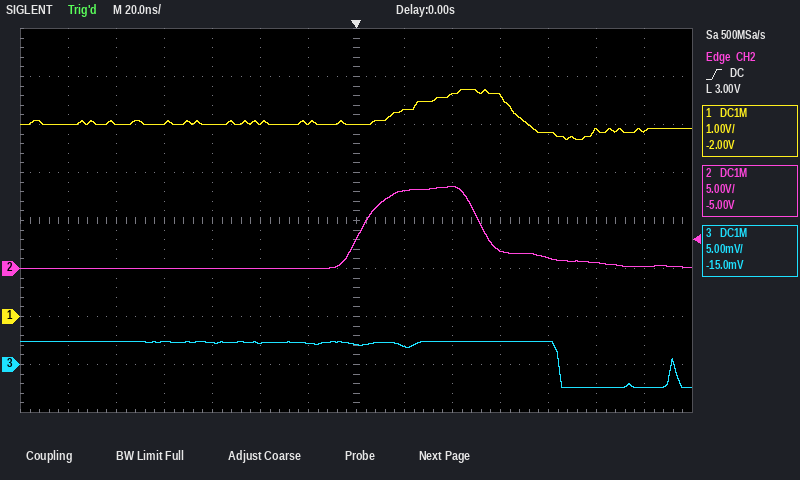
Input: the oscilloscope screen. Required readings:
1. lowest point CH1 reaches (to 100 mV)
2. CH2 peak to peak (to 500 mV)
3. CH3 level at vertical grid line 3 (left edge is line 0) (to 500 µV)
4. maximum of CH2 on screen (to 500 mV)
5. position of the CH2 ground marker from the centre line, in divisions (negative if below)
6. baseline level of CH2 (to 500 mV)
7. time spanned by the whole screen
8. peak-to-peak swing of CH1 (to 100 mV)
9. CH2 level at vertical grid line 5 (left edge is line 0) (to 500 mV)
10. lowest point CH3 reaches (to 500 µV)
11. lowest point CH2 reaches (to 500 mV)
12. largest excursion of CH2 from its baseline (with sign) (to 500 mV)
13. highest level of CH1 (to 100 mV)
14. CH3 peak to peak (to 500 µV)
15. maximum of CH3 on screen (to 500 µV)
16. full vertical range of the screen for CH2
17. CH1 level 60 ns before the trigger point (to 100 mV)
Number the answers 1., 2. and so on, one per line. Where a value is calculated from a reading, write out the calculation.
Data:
1. 3.7 V
2. 8.5 V − (0.0 V) = 8.5 V
3. 2.5 mV
4. 8.5 V
5. -1.0 div
6. 0.0 V
7. 280 ns
8. 4.7 V − (3.7 V) = 1.0 V
9. 0.0 V
10. -2.5 mV
11. 0.0 V
12. 8.5 V − (0.0 V) = +8.5 V
13. 4.7 V
14. 2.5 mV − (-2.5 mV) = 5.0 mV
15. 2.5 mV
16. 40 V
17. 4.0 V
